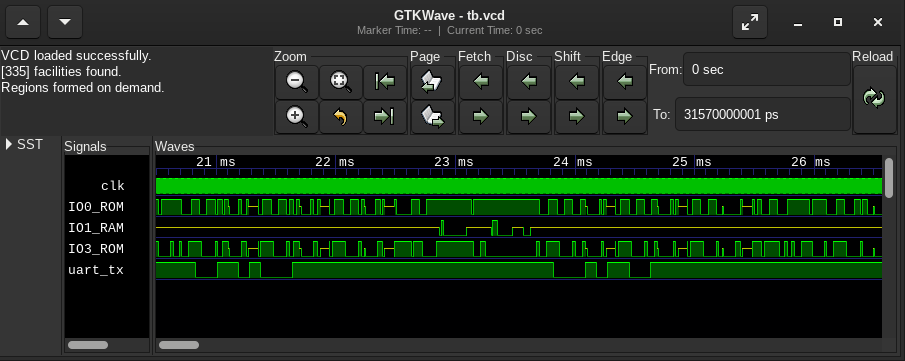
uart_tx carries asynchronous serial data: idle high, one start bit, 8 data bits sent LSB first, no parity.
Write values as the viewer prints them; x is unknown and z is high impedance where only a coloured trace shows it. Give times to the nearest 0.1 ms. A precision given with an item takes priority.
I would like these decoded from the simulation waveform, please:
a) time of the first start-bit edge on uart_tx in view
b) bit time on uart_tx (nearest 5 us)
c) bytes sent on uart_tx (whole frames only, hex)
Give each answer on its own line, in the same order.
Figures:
20.8 ms
90 us
16, 34
